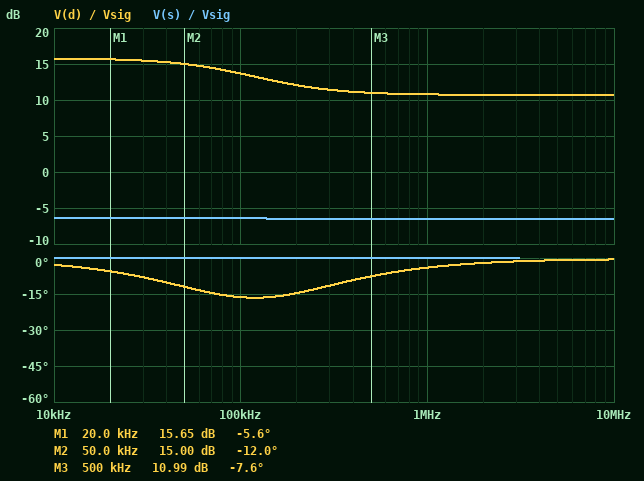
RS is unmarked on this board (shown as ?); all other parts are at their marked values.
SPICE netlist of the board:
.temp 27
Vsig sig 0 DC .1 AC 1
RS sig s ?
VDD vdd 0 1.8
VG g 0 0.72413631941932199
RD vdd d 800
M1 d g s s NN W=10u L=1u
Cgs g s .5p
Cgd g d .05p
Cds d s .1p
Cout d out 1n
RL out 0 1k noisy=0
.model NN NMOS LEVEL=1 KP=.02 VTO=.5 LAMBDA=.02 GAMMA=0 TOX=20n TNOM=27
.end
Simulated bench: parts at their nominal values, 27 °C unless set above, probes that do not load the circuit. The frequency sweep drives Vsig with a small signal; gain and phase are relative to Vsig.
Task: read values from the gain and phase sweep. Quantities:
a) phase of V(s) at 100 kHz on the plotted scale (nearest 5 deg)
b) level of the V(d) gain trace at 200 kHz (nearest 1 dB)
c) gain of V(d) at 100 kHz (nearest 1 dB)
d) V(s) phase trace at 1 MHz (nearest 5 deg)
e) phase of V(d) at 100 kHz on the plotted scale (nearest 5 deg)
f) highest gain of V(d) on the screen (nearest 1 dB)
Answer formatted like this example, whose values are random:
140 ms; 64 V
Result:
0 deg; 12 dB; 14 dB; 0 deg; -15 deg; 16 dB
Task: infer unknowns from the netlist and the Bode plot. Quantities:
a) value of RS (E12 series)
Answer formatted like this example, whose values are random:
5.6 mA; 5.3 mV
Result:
68 Ω
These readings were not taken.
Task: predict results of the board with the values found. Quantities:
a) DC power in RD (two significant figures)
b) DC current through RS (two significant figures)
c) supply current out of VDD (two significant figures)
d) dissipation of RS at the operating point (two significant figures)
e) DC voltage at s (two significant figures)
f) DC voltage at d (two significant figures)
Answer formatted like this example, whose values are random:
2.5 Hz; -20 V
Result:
340 µW; 650 µA; 650 µA; 29 µW; 140 mV; 1.3 V
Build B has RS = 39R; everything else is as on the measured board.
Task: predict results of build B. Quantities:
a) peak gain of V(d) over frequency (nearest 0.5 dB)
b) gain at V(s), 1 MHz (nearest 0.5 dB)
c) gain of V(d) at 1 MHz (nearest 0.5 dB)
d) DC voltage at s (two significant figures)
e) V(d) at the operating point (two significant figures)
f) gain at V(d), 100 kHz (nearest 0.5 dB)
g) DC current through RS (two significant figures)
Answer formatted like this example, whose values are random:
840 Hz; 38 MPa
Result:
18.5 dB; -4.5 dB; 13.5 dB; 130 mV; 1.1 V; 16.5 dB; 850 µA
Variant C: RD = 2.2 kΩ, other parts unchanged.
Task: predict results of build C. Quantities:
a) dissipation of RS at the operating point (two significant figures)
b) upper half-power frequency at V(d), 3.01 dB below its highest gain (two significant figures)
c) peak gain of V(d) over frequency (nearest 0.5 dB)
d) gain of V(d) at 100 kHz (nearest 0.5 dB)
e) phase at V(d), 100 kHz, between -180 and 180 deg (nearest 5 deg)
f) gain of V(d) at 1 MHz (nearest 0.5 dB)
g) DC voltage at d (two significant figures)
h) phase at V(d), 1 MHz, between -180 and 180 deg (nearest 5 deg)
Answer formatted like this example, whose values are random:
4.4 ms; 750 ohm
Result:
28 µW; 56 kHz; 24.5 dB; 19.0 dB; -30 deg; 14.5 dB; 380 mV; -5 deg
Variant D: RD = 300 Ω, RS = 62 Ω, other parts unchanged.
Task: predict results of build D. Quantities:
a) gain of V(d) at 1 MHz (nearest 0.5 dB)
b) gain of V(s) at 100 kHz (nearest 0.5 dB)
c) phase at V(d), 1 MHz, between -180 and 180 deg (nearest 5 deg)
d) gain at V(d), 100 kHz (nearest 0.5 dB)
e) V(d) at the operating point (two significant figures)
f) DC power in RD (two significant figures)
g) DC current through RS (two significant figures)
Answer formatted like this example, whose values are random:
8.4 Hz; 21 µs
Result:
5.5 dB; -6.0 dB; 0 deg; 7.0 dB; 1.6 V; 140 µW; 690 µA
